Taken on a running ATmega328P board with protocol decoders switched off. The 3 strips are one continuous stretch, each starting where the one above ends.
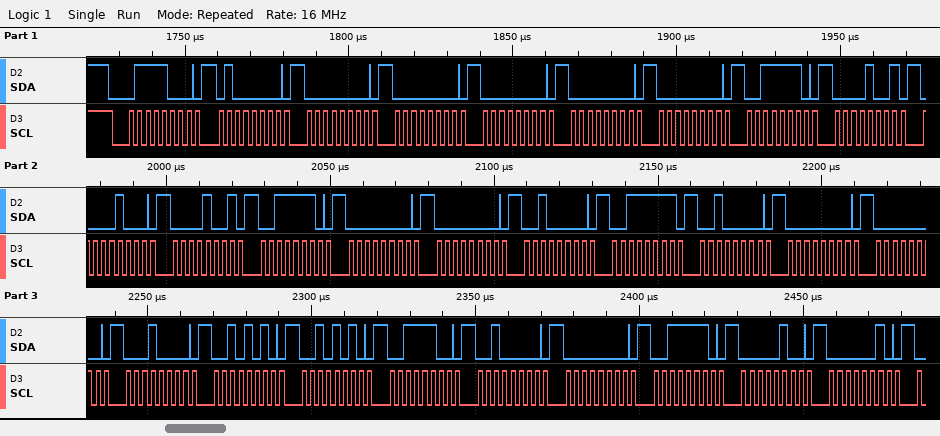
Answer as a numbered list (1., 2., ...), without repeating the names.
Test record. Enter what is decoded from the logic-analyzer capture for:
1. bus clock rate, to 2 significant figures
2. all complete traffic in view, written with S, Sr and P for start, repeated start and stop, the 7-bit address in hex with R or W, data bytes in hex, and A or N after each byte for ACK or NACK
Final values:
1. 400 kHz
2. S 3CW A 40 A 00 A 00 A 00 A 00 A 00 A 3E A 09 A 08 A 09 A 3E A 00 A 00 A 20 A 3F A 20 A 00 A 00 A 10 A 2A A 2A A 3C A 20 A 00 A 3E A 04 A 02 A
